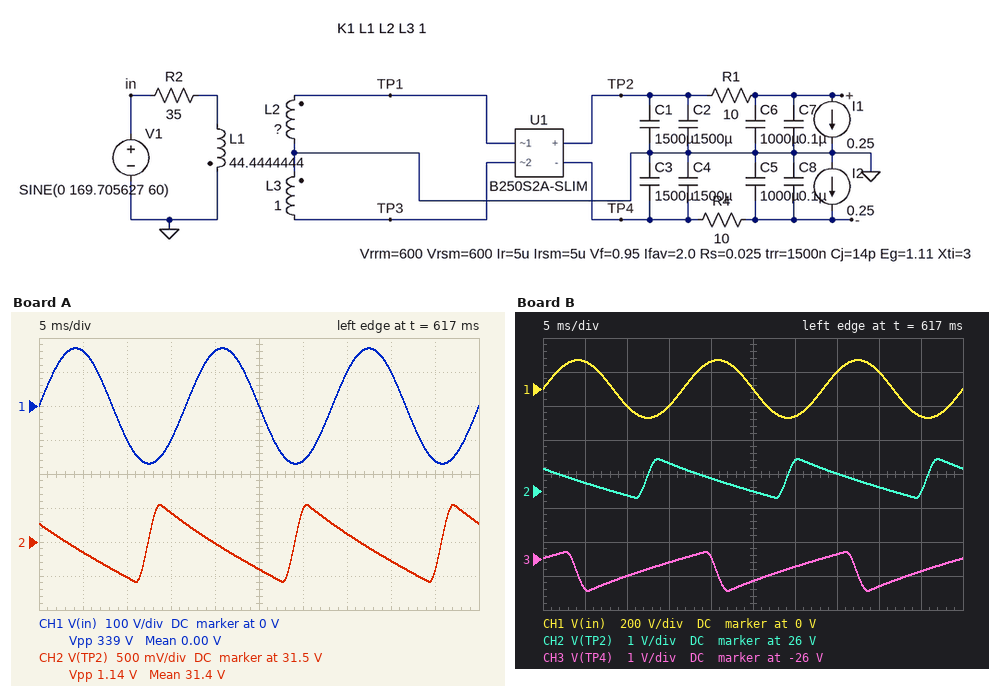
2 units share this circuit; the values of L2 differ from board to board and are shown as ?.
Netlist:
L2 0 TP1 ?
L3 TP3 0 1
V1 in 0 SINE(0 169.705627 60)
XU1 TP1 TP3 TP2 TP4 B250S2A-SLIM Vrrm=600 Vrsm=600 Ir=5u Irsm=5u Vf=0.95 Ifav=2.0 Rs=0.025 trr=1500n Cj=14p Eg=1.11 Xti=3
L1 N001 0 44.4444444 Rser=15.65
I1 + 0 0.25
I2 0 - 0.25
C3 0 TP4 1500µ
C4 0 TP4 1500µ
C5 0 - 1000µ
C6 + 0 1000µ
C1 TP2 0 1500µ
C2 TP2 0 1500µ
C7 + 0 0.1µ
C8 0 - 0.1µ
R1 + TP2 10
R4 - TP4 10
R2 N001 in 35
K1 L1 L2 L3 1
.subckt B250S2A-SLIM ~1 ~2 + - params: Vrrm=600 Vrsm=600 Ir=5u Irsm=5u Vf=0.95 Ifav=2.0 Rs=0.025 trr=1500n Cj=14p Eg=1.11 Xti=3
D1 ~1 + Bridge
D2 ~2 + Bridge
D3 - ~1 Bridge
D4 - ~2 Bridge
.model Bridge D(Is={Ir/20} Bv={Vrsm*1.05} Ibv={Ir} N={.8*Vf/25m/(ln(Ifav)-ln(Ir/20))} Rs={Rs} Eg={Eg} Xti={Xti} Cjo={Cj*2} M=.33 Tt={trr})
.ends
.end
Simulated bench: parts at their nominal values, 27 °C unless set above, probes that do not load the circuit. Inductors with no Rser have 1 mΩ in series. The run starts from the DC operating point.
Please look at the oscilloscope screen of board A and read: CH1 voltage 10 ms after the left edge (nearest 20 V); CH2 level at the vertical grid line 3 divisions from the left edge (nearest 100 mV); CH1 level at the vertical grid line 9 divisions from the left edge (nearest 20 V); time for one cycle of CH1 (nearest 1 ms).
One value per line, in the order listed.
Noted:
-100 V
31.9 V
-160 V
17 ms
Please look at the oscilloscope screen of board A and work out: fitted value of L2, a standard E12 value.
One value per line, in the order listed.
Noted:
2.2 H
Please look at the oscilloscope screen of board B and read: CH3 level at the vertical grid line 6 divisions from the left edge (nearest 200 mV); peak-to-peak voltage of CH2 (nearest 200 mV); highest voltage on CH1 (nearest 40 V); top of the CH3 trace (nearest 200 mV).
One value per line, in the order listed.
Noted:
-26.2 V
1.2 V
160 V
-25.8 V
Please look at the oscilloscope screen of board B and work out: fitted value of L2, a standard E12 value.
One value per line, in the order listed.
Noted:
1.5 H
